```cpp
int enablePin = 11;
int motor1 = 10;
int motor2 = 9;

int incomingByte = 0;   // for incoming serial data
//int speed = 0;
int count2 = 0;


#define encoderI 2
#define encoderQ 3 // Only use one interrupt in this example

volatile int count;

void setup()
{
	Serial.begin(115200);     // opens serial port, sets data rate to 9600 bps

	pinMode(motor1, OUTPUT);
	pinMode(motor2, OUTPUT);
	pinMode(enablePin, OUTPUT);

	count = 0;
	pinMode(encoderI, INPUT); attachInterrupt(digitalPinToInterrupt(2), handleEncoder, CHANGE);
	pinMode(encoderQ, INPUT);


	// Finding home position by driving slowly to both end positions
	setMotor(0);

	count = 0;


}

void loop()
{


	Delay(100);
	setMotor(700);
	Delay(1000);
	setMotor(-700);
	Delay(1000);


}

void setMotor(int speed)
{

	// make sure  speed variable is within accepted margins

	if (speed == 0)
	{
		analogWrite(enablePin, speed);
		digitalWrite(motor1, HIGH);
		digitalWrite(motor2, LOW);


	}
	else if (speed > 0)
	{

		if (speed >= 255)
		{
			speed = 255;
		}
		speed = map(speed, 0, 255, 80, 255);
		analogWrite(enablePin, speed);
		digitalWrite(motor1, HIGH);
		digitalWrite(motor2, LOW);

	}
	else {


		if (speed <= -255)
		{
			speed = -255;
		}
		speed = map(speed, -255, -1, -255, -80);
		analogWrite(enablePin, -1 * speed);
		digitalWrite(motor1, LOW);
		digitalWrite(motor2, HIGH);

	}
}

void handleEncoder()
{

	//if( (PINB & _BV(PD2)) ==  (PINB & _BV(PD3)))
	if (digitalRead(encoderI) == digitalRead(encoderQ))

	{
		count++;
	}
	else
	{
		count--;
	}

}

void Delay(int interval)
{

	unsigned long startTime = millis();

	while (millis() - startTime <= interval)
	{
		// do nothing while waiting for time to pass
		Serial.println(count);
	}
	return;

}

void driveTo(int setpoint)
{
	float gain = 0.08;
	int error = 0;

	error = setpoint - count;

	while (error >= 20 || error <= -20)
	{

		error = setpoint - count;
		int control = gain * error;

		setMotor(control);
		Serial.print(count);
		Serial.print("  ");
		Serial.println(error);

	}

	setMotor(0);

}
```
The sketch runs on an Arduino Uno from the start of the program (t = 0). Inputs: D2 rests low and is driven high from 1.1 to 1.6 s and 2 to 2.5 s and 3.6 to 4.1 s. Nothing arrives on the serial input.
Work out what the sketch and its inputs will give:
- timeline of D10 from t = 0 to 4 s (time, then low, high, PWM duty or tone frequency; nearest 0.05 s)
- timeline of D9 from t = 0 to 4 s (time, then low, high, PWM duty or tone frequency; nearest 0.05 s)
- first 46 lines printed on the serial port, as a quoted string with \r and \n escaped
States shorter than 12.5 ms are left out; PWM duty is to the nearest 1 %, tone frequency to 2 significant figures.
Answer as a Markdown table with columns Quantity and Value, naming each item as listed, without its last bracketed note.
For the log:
| Quantity | Value |
|---|---|
| timeline of D10 from t = 0 to 4 s | 0 s high; 1.1 s low; 2.2 s high; 3.2 s low |
| timeline of D9 from t = 0 to 4 s | 0 s low; 1.1 s high; 2.2 s low; 3.2 s high |
| first 46 lines printed on the serial port, as a quoted string with \r and \n escaped | "0\r\n0\r\n0\r\n0\r\n0\r\n0\r\n0\r\n0\r\n0\r\n0\r\n0\r\n0\r\n0\r\n0\r\n0\r\n0\r\n0\r\n0\r\n0\r\n0\r\n0\r\n0\r\n0\r\n0\r\n0\r\n0\r\n0\r\n0\r\n0\r\n0\r\n0\r\n0\r\n0\r\n0\r\n0\r\n0\r\n0\r\n0\r\n0\r\n0\r\n0\r\n0\r\n0\r\n0\r\n0\r\n0\r\n" |
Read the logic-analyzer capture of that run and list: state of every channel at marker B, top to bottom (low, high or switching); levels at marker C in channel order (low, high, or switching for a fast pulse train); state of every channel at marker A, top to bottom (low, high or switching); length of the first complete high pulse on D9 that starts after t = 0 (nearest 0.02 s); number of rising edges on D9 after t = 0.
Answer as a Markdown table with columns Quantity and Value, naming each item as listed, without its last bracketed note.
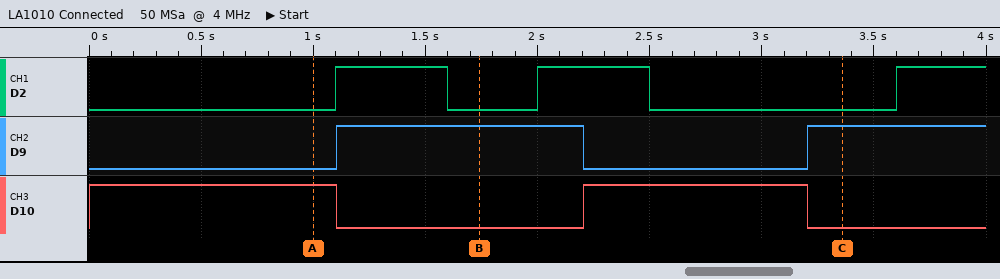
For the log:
| Quantity | Value |
|---|---|
| state of every channel at marker B, top to bottom | D2 low, D9 high, D10 low |
| levels at marker C in channel order | D2 low, D9 high, D10 low |
| state of every channel at marker A, top to bottom | D2 low, D9 low, D10 high |
| length of the first complete high pulse on D9 that starts after t = 0 | 1.10 s |
| number of rising edges on D9 after t = 0 | 2 |
